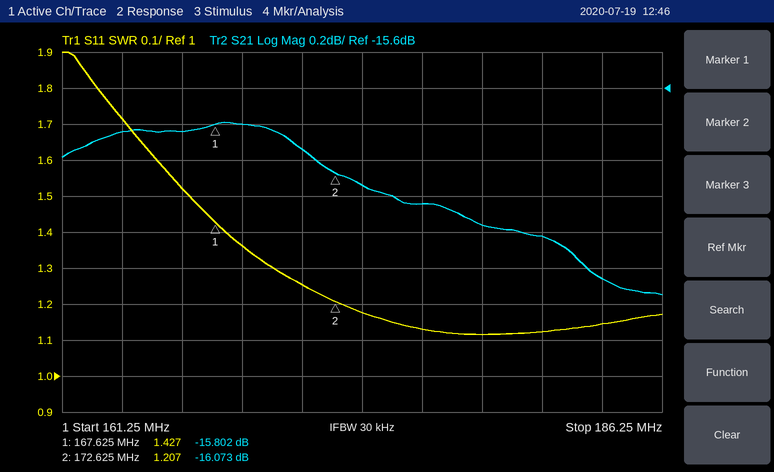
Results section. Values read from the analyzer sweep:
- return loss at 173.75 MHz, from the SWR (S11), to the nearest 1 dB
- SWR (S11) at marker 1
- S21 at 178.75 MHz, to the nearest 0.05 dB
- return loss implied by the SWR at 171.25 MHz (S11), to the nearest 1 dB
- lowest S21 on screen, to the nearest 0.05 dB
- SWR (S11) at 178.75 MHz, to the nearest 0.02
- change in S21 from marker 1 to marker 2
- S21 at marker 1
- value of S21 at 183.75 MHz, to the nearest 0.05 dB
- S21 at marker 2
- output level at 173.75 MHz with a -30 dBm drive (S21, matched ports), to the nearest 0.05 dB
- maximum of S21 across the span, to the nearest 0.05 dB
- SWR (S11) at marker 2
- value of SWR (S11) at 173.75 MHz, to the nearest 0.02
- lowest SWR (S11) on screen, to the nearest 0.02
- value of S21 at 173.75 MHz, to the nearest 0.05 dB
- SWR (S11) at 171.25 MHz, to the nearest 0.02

22 dB
1.427
-16.35 dB
19 dB
-16.75 dB
1.12
-0.271 dB
-15.802 dB
-16.65 dB
-16.073 dB
-46.15 dBm
-15.80 dB
1.207
1.18
1.12
-16.15 dB
1.26
